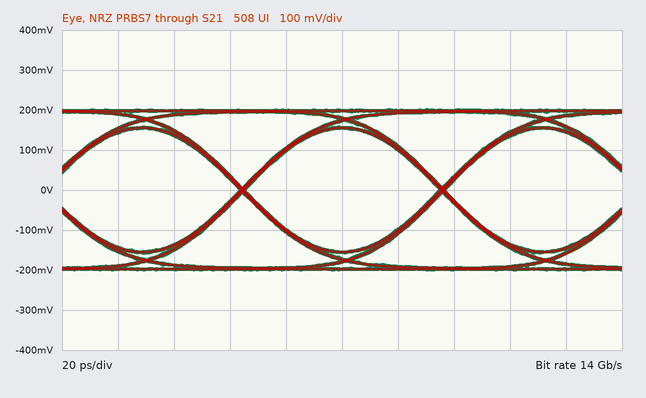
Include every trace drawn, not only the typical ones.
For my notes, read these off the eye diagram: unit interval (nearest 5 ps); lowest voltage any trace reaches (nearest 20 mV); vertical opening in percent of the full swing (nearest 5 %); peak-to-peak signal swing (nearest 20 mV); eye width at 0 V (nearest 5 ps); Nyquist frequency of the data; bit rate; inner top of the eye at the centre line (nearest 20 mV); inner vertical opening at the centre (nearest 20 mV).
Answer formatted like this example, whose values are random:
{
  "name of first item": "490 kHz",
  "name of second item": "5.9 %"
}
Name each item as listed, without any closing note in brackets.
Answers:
{
  "unit interval": "70 ps",
  "lowest voltage any trace reaches": "-200 mV",
  "vertical opening in percent of the full swing": "75 %",
  "peak-to-peak signal swing": "400 mV",
  "eye width at 0 V": "70 ps",
  "Nyquist frequency of the data": "7 GHz",
  "bit rate": "14 Gb/s",
  "inner top of the eye at the centre line": "160 mV",
  "inner vertical opening at the centre": "300 mV"
}
